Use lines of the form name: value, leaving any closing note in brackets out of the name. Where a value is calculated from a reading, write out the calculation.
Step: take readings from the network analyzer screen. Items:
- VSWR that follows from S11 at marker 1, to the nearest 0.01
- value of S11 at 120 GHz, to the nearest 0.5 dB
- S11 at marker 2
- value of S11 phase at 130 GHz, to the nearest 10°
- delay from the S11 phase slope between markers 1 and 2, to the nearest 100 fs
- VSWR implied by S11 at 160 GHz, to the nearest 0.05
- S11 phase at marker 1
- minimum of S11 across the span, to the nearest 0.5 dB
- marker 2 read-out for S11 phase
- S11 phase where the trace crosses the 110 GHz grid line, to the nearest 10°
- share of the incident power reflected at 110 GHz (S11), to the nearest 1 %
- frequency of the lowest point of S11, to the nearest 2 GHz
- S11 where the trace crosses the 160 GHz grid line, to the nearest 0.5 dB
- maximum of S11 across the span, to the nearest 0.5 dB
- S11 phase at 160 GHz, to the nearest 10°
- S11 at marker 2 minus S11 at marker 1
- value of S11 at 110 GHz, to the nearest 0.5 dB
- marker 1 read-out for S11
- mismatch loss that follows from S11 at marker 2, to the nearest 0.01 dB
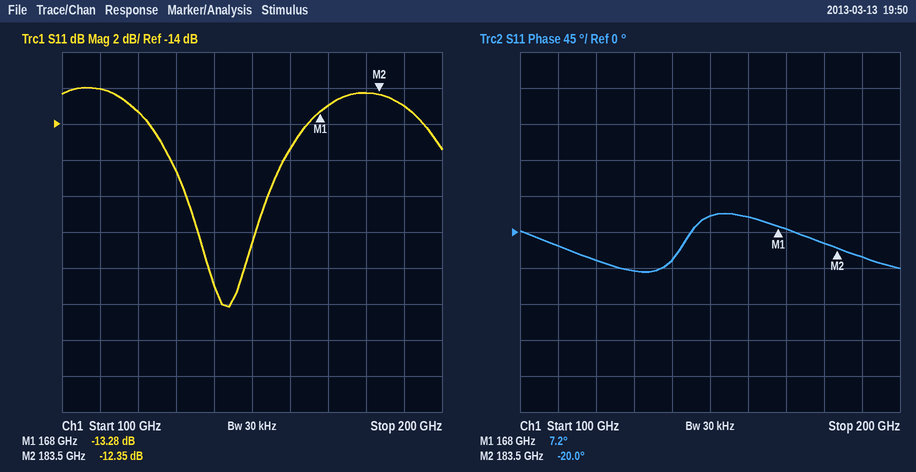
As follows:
VSWR that follows from S11 at marker 1, to the nearest 0.01: (1 + 0.2168)/(1 − 0.2168) ≈ 1.55
value of S11 at 120 GHz, to the nearest 0.5 dB: -13.5 dB
S11 at marker 2: -12.35 dB
value of S11 phase at 130 GHz, to the nearest 10°: -50°
delay from the S11 phase slope between markers 1 and 2, to the nearest 100 fs: −(-20° − (7.2°))/(360° × 15.5 GHz) ≈ 4.9 ps
VSWR implied by S11 at 160 GHz, to the nearest 0.05: |Γ| = 10^(-15.5/20) = 0.1679; VSWR = (1 + 0.1679)/(1 − 0.1679) ≈ 1.40
S11 phase at marker 1: 7.2°
minimum of S11 across the span, to the nearest 0.5 dB: -24.0 dB
marker 2 read-out for S11 phase: -20.0°
S11 phase where the trace crosses the 110 GHz grid line, to the nearest 10°: -20°
share of the incident power reflected at 110 GHz (S11), to the nearest 1 %: 10^(-12/10) ≈ 6 %
frequency of the lowest point of S11, to the nearest 2 GHz: 144 GHz
S11 where the trace crosses the 160 GHz grid line, to the nearest 0.5 dB: -15.5 dB
maximum of S11 across the span, to the nearest 0.5 dB: -12.0 dB
S11 phase at 160 GHz, to the nearest 10°: 20°
S11 at marker 2 minus S11 at marker 1: -12.35 − (-13.28) = 0.93 dB
value of S11 at 110 GHz, to the nearest 0.5 dB: -12.0 dB
marker 1 read-out for S11: -13.28 dB
mismatch loss that follows from S11 at marker 2, to the nearest 0.01 dB: −10 log10(1 − 10^(-12.35/10)) ≈ 0.26 dB
